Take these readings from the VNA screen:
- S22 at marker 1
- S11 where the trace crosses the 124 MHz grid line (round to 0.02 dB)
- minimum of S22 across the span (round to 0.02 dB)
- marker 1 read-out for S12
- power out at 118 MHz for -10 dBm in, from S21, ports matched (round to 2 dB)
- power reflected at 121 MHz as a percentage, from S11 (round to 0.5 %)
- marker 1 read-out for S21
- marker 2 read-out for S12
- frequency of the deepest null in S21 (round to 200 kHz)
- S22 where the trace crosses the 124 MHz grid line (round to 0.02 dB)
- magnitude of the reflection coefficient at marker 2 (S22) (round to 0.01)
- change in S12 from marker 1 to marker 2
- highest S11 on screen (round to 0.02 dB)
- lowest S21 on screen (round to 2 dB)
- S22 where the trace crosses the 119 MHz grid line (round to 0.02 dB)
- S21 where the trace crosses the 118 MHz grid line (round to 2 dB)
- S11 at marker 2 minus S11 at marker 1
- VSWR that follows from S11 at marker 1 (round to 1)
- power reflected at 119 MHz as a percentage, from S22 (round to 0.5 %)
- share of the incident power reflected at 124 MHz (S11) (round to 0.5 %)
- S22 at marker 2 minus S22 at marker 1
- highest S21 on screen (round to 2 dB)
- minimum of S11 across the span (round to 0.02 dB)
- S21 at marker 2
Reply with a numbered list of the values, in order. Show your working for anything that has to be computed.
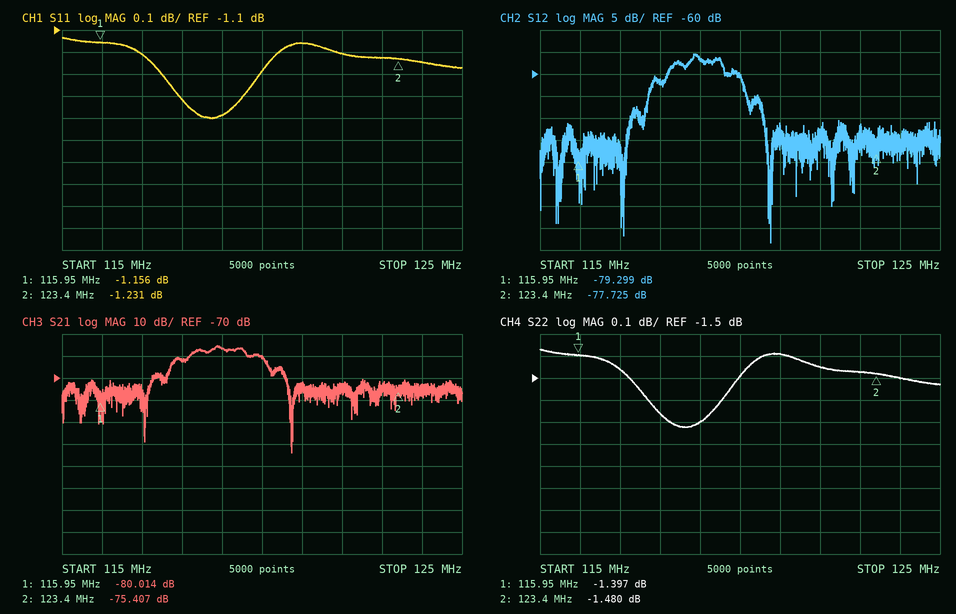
1. -1.397 dB
2. -1.24 dB
3. -1.72 dB
4. -79.299 dB
5. -10 dBm + (-62 dB) = -72 dBm
6. 10^(-1.16/10) ≈ 76.6 %, so 76.5 % to the nearest 0.5 %
7. -80.014 dB
8. -77.725 dB
9. 120.8 MHz
10. -1.50 dB
11. 10^(-1.48/20) ≈ 0.84
12. -77.725 − (-79.299) = 1.574 dB
13. -1.14 dB
14. -104 dB
15. -1.70 dB
16. -62 dB
17. -1.231 − (-1.156) = -0.075 dB
18. (1 + 0.8754)/(1 − 0.8754) ≈ 15
19. 10^(-1.7/10) ≈ 67.6 %, so 67.5 % to the nearest 0.5 %
20. 10^(-1.24/10) ≈ 75.2 %, so 75.0 % to the nearest 0.5 %
21. -1.48 − (-1.397) = -0.083 dB
22. -56 dB
23. -1.50 dB
24. -75.407 dB
